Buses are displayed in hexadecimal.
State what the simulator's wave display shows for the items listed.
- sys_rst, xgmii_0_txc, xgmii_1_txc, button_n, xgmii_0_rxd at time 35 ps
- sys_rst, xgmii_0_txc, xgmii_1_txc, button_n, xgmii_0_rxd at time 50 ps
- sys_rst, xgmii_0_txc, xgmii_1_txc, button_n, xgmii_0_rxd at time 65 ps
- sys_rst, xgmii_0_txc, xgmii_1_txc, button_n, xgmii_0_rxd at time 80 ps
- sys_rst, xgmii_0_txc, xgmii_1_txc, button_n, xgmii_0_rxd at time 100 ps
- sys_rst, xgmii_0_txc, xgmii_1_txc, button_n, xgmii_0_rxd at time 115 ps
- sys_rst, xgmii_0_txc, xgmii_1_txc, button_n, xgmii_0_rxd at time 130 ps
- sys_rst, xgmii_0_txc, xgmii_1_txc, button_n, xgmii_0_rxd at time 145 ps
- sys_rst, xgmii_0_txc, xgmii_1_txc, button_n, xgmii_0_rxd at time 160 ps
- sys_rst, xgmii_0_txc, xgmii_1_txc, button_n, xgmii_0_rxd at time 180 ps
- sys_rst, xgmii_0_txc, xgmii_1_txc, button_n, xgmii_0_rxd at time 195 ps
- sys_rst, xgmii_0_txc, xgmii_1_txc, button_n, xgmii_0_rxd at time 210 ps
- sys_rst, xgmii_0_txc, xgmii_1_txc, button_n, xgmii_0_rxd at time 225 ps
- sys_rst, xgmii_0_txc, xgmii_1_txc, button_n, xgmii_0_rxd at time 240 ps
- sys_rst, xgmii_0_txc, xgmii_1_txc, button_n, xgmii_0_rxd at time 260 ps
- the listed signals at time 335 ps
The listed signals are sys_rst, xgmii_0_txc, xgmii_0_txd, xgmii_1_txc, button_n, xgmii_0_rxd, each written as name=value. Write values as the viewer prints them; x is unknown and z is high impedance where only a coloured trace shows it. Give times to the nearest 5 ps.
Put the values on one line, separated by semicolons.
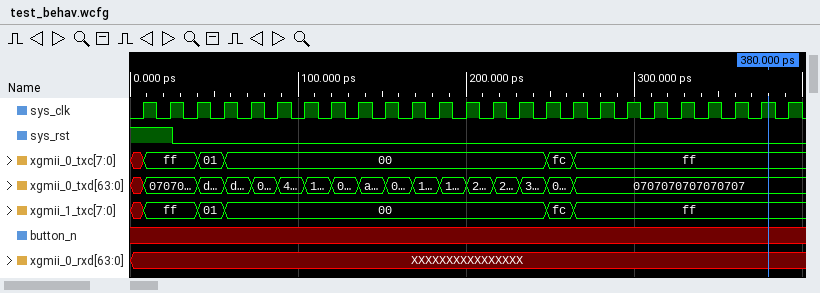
sys_rst=0, xgmii_0_txc=ff, xgmii_1_txc=ff, button_n=x, xgmii_0_rxd=XXXXXXXXXXXXXXXX; sys_rst=0, xgmii_0_txc=01, xgmii_1_txc=01, button_n=x, xgmii_0_rxd=XXXXXXXXXXXXXXXX; sys_rst=0, xgmii_0_txc=00, xgmii_1_txc=00, button_n=x, xgmii_0_rxd=XXXXXXXXXXXXXXXX; sys_rst=0, xgmii_0_txc=00, xgmii_1_txc=00, button_n=x, xgmii_0_rxd=XXXXXXXXXXXXXXXX; sys_rst=0, xgmii_0_txc=00, xgmii_1_txc=00, button_n=x, xgmii_0_rxd=XXXXXXXXXXXXXXXX; sys_rst=0, xgmii_0_txc=00, xgmii_1_txc=00, button_n=x, xgmii_0_rxd=XXXXXXXXXXXXXXXX; sys_rst=0, xgmii_0_txc=00, xgmii_1_txc=00, button_n=x, xgmii_0_rxd=XXXXXXXXXXXXXXXX; sys_rst=0, xgmii_0_txc=00, xgmii_1_txc=00, button_n=x, xgmii_0_rxd=XXXXXXXXXXXXXXXX; sys_rst=0, xgmii_0_txc=00, xgmii_1_txc=00, button_n=x, xgmii_0_rxd=XXXXXXXXXXXXXXXX; sys_rst=0, xgmii_0_txc=00, xgmii_1_txc=00, button_n=x, xgmii_0_rxd=XXXXXXXXXXXXXXXX; sys_rst=0, xgmii_0_txc=00, xgmii_1_txc=00, button_n=x, xgmii_0_rxd=XXXXXXXXXXXXXXXX; sys_rst=0, xgmii_0_txc=00, xgmii_1_txc=00, button_n=x, xgmii_0_rxd=XXXXXXXXXXXXXXXX; sys_rst=0, xgmii_0_txc=00, xgmii_1_txc=00, button_n=x, xgmii_0_rxd=XXXXXXXXXXXXXXXX; sys_rst=0, xgmii_0_txc=00, xgmii_1_txc=00, button_n=x, xgmii_0_rxd=XXXXXXXXXXXXXXXX; sys_rst=0, xgmii_0_txc=fc, xgmii_1_txc=fc, button_n=x, xgmii_0_rxd=XXXXXXXXXXXXXXXX; sys_rst=0, xgmii_0_txc=ff, xgmii_0_txd=0707070707070707, xgmii_1_txc=ff, button_n=x, xgmii_0_rxd=XXXXXXXXXXXXXXXX
